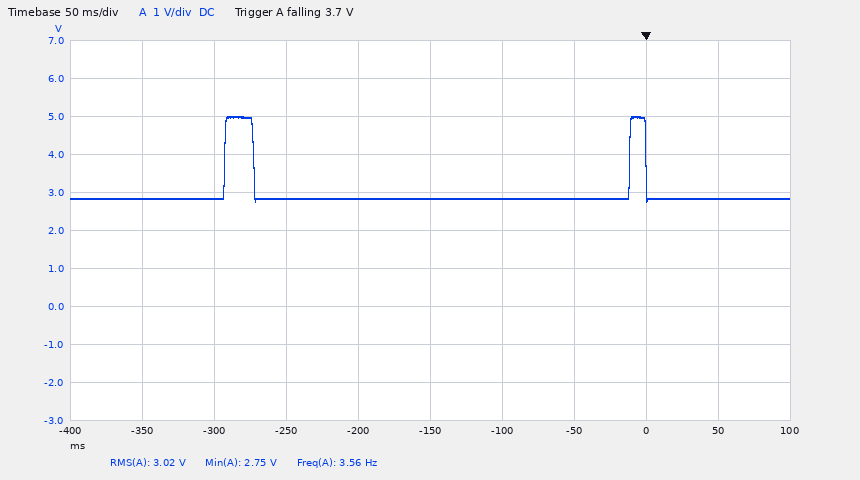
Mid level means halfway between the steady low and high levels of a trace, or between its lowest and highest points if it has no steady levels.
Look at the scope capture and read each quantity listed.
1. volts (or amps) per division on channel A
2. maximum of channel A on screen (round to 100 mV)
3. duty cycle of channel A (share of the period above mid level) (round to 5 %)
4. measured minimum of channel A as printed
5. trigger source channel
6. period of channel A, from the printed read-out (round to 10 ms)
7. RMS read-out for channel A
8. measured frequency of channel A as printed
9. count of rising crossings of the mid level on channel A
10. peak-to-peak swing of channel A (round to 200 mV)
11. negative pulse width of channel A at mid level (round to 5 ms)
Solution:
1 V
5.0 V
5 %
2.75 V
channel A
280 ms
3.02 V
3.56 Hz
2
2.2 V
265 ms
